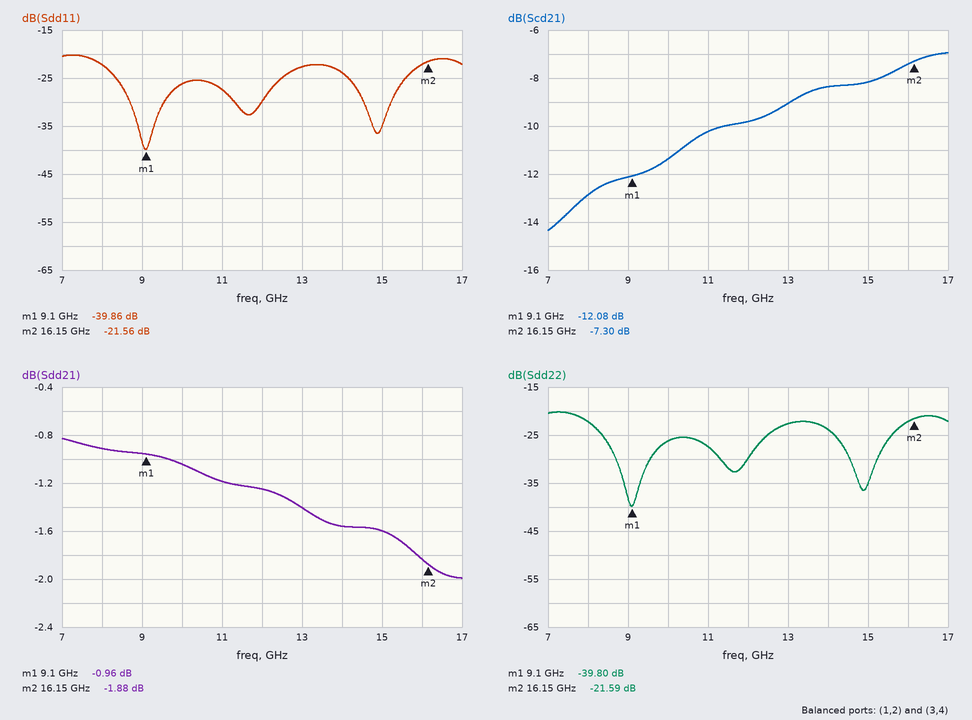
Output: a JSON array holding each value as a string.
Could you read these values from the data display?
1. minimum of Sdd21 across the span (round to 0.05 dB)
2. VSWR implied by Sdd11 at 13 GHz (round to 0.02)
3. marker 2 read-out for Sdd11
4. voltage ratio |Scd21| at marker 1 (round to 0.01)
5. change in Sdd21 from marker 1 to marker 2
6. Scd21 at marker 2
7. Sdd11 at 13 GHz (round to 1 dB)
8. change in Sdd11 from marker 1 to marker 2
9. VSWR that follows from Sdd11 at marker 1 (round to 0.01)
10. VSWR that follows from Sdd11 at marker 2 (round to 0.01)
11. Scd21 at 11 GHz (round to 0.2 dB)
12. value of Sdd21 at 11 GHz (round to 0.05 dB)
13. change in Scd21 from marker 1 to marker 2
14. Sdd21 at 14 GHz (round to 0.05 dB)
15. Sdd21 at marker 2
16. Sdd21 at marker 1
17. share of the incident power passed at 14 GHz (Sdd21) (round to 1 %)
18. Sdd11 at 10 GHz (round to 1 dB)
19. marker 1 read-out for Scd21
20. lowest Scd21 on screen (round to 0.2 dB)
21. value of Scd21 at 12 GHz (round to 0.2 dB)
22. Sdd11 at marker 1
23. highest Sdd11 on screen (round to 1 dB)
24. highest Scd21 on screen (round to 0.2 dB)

["-2.00 dB", "1.16", "-21.56 dB", "0.25", "-0.92 dB", "-7.30 dB", "-23 dB", "18.30 dB", "1.02", "1.18", "-10.2 dB", "-1.20 dB", "4.78 dB", "-1.55 dB", "-1.88 dB", "-0.96 dB", "70 %", "-26 dB", "-12.08 dB", "-14.4 dB", "-9.8 dB", "-39.86 dB", "-20 dB", "-7.0 dB"]
